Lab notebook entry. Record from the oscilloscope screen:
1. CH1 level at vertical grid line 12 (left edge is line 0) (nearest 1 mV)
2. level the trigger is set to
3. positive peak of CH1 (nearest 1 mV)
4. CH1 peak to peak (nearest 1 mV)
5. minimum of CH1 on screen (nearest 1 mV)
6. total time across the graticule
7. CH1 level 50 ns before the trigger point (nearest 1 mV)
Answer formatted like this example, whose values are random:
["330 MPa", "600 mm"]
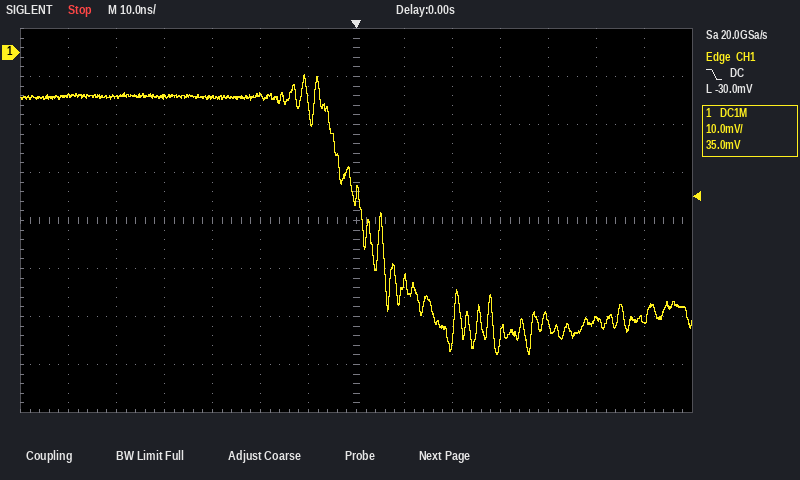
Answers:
["-55 mV", "-30.0 mV", "-5 mV", "58 mV", "-63 mV", "140 ns", "-9 mV"]
